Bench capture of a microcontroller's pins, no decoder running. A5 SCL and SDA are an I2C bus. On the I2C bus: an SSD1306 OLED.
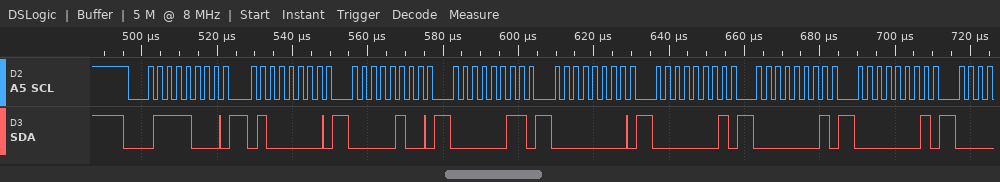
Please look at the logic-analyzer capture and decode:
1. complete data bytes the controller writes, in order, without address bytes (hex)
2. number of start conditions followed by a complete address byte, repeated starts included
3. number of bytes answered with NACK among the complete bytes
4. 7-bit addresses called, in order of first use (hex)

40 04 03 00 01 01 01
1
0
0x3C
